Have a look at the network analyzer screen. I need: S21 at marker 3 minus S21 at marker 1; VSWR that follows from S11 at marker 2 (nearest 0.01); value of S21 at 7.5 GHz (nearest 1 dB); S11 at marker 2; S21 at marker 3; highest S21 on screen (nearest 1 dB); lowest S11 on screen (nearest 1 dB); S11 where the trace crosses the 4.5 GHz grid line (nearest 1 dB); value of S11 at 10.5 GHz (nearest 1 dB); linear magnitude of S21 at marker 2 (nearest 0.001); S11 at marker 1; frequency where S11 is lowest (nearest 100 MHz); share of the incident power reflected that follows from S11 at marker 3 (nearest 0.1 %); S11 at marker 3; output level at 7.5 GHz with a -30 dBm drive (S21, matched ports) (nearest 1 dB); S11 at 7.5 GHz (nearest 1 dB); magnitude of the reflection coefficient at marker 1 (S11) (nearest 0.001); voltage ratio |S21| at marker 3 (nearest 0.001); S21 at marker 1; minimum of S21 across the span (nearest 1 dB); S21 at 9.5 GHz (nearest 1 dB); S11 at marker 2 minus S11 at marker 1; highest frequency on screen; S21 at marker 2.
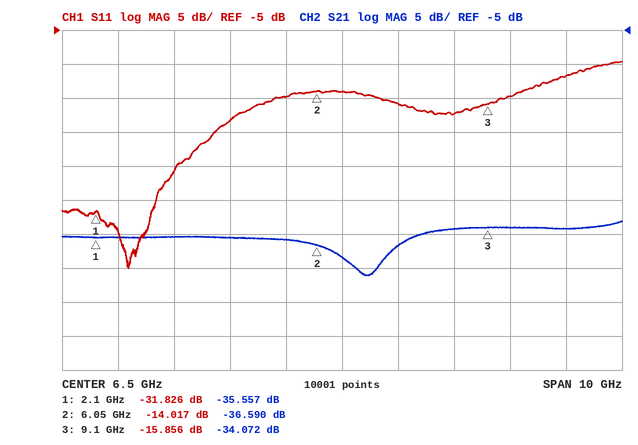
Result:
1.485 dB
1.50
-37 dB
-14.017 dB
-34.072 dB
-33 dB
-40 dB
-18 dB
-12 dB
0.015
-31.826 dB
2.7 GHz
2.6 %
-15.856 dB
-67 dBm
-16 dB
0.026
0.020
-35.557 dB
-41 dB
-34 dB
17.809 dB
11.5 GHz
-36.590 dB
